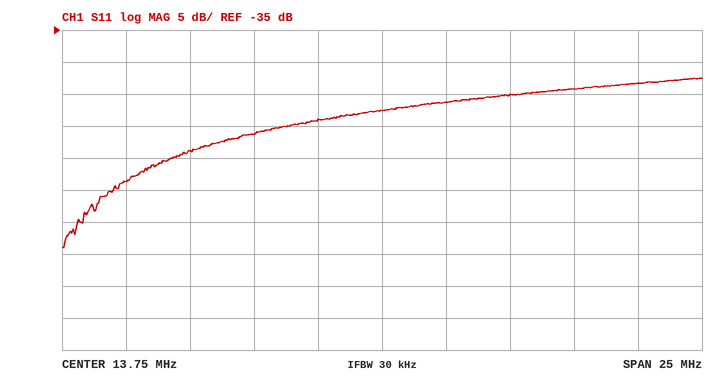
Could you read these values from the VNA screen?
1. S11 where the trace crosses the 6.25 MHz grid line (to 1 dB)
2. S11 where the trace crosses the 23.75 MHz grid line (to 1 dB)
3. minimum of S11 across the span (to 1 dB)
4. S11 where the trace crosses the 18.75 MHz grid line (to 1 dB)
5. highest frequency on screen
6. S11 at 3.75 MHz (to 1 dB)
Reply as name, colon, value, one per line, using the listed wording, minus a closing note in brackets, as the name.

S11 where the trace crosses the 6.25 MHz grid line: -54 dB
S11 where the trace crosses the 23.75 MHz grid line: -43 dB
minimum of S11 across the span: -69 dB
S11 where the trace crosses the 18.75 MHz grid line: -45 dB
highest frequency on screen: 26.25 MHz
S11 at 3.75 MHz: -59 dB
